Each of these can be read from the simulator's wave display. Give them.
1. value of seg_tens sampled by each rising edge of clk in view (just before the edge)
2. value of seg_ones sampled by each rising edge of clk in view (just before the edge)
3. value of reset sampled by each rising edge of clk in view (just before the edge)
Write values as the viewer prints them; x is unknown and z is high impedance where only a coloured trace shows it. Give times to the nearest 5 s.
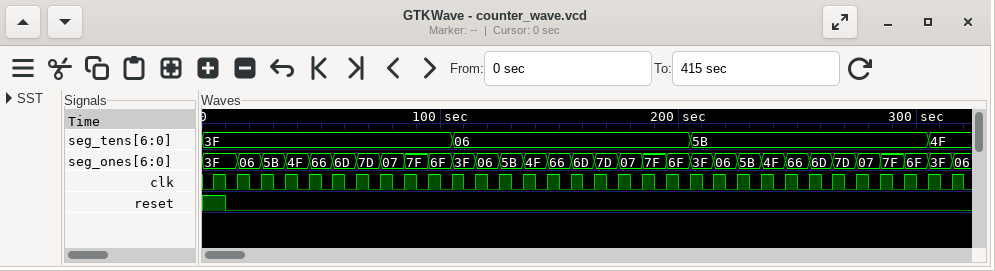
3F, 3F, 3F, 3F, 3F, 3F, 3F, 3F, 3F, 3F, 3F, 06, 06, 06, 06, 06, 06, 06, 06, 06, 06, 5B, 5B, 5B, 5B, 5B, 5B, 5B, 5B, 5B, 5B, 4F
3F, 3F, 06, 5B, 4F, 66, 6D, 7D, 07, 7F, 6F, 3F, 06, 5B, 4F, 66, 6D, 7D, 07, 7F, 6F, 3F, 06, 5B, 4F, 66, 6D, 7D, 07, 7F, 6F, 3F
1 0 0 0 0 0 0 0 0 0 0 0 0 0 0 0 0 0 0 0 0 0 0 0 0 0 0 0 0 0 0 0
